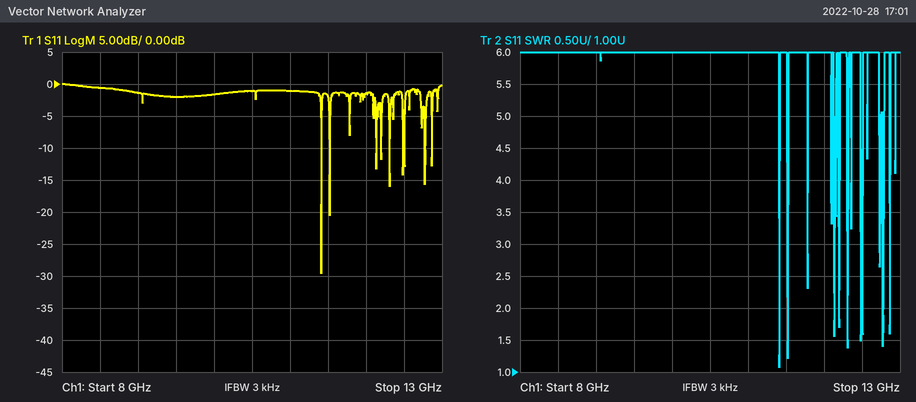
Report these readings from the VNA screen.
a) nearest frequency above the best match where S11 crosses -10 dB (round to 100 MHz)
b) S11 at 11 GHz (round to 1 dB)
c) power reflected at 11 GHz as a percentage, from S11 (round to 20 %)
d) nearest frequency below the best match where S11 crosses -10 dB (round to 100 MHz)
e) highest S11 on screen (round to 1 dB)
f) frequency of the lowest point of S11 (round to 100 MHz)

11.4 GHz
-1 dB
80 %
11.4 GHz
0 dB
11.4 GHz
